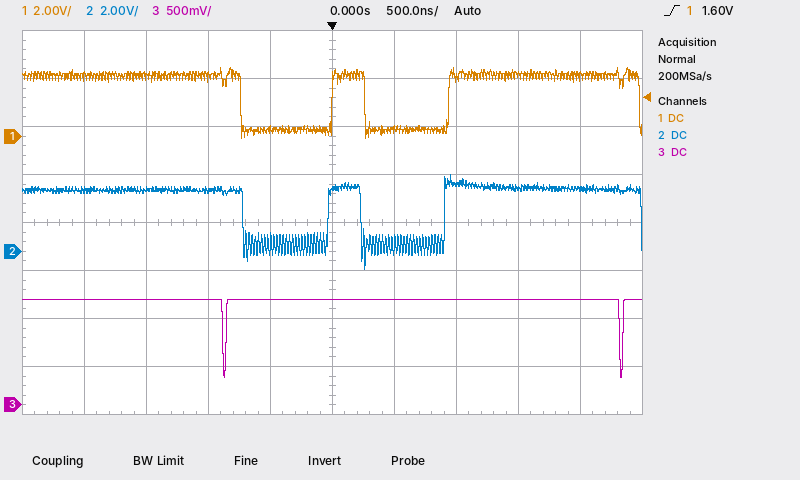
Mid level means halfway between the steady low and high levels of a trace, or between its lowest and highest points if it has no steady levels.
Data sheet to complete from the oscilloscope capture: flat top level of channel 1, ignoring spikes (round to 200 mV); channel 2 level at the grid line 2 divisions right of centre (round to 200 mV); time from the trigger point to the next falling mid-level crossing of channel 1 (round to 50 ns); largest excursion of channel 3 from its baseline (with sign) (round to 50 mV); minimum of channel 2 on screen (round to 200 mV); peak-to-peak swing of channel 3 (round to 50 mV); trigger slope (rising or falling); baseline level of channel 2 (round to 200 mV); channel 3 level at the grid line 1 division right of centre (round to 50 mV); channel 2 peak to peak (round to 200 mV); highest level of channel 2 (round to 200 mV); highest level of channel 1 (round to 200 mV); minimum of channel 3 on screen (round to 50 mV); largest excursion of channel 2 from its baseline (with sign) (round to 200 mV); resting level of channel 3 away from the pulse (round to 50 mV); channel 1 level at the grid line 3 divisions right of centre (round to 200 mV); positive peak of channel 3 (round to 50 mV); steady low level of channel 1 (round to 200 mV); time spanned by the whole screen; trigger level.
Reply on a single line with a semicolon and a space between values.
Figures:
2.6 V; 2.8 V; 250 ns; -800 mV; -800 mV; 800 mV; rising; 2.6 V; 1.10 V; 4.0 V; 3.2 V; 2.8 V; 300 mV; -3.4 V; 1.10 V; 2.6 V; 1.10 V; 200 mV; 5 µs; 1.60 V
